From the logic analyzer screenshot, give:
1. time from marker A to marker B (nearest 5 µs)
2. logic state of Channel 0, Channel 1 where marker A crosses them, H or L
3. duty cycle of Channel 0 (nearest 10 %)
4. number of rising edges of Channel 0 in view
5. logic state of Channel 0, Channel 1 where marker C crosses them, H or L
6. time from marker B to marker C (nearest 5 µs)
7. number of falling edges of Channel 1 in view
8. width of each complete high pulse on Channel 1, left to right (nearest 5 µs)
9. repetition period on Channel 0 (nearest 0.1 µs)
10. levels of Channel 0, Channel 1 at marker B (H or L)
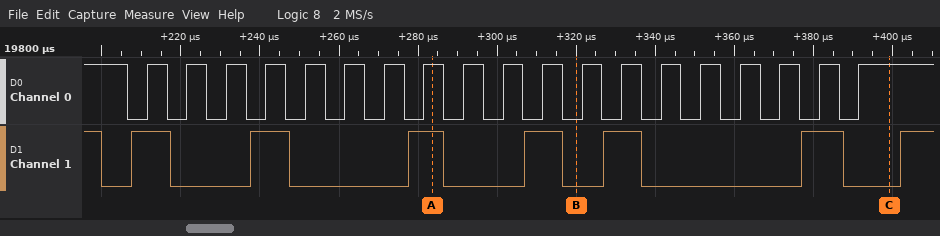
35 µs
Channel 0=H, Channel 1=H
50 %
19
Channel 0=H, Channel 1=L
80 µs
7
10 µs, 10 µs, 10 µs, 10 µs, 10 µs, 10 µs
10 µs
Channel 0=L, Channel 1=L
